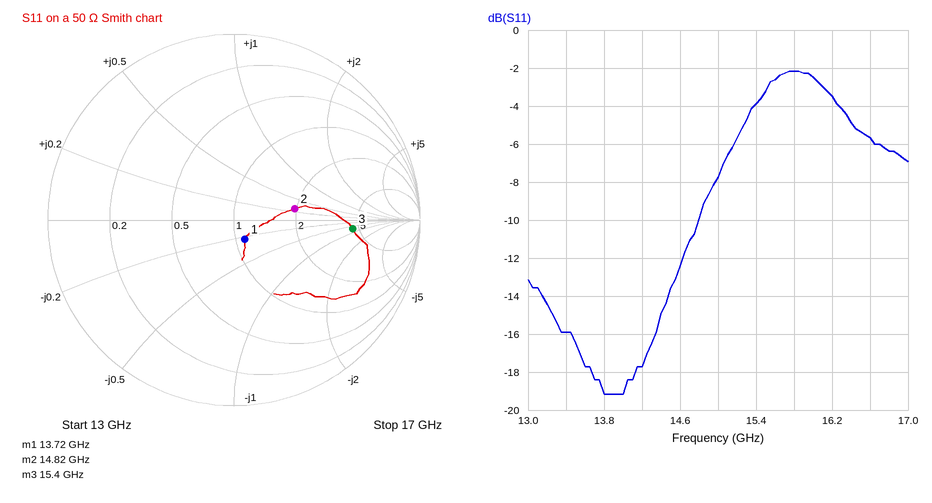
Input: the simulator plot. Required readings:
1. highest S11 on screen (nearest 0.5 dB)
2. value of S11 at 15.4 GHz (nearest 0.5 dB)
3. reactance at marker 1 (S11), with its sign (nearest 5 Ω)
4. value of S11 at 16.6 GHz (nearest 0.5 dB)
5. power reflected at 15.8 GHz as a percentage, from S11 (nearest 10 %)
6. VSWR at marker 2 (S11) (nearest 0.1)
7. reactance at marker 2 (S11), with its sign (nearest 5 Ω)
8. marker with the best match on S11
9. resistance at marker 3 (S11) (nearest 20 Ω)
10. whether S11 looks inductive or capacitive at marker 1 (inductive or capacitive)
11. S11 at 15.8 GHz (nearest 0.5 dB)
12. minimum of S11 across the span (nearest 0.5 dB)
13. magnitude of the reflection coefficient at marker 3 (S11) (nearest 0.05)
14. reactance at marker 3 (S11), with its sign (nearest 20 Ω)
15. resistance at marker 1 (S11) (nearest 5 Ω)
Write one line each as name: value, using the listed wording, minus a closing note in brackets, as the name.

highest S11 on screen: -2.0 dB
value of S11 at 15.4 GHz: -4.0 dB
reactance at marker 1 (S11), with its sign: -10 Ω
value of S11 at 16.6 GHz: -5.5 dB
power reflected at 15.8 GHz as a percentage, from S11: 60 %
VSWR at marker 2 (S11): 2.0
reactance at marker 2 (S11), with its sign: +15 Ω
marker with the best match on S11: marker 1
resistance at marker 3 (S11): 220 Ω
whether S11 looks inductive or capacitive at marker 1: capacitive
S11 at 15.8 GHz: -2.0 dB
minimum of S11 across the span: -19.0 dB
magnitude of the reflection coefficient at marker 3 (S11): 0.65
reactance at marker 3 (S11), with its sign: -40 Ω
resistance at marker 1 (S11): 55 Ω
